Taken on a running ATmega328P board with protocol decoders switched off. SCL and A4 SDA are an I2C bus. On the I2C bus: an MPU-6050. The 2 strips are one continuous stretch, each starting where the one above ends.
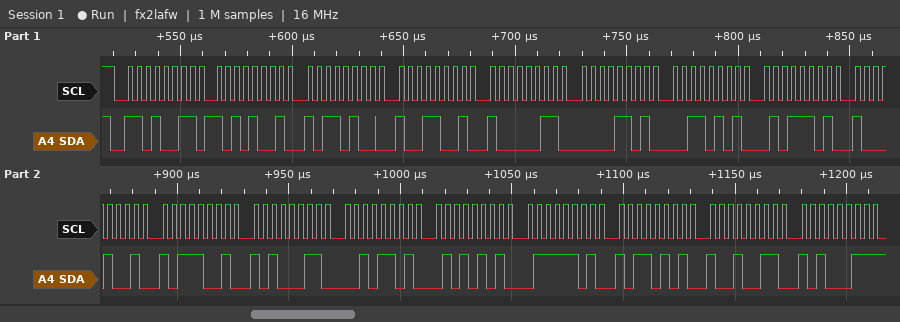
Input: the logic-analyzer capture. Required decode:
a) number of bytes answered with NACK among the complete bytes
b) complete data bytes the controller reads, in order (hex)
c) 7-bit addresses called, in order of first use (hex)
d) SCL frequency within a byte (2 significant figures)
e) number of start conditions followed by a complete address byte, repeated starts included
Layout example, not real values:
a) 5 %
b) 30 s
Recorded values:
a) 1
b) A9 B4 99 83 0D 35 5D 89 B9 A3 2D 55 7D B5 93 A3
c) 0x69
d) 250 kHz
e) 1
